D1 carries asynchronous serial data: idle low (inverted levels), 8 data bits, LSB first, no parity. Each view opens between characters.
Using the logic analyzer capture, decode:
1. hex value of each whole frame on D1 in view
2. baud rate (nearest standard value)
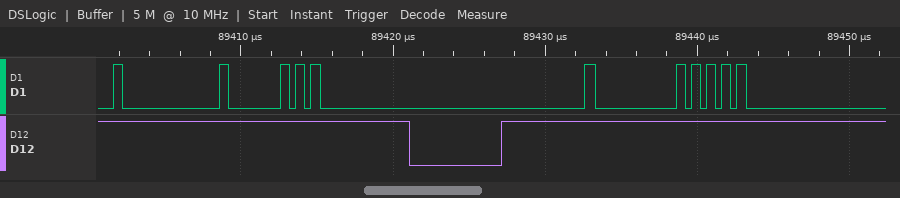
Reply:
FF, 7F, FD, FF, 55
2000000 baud
